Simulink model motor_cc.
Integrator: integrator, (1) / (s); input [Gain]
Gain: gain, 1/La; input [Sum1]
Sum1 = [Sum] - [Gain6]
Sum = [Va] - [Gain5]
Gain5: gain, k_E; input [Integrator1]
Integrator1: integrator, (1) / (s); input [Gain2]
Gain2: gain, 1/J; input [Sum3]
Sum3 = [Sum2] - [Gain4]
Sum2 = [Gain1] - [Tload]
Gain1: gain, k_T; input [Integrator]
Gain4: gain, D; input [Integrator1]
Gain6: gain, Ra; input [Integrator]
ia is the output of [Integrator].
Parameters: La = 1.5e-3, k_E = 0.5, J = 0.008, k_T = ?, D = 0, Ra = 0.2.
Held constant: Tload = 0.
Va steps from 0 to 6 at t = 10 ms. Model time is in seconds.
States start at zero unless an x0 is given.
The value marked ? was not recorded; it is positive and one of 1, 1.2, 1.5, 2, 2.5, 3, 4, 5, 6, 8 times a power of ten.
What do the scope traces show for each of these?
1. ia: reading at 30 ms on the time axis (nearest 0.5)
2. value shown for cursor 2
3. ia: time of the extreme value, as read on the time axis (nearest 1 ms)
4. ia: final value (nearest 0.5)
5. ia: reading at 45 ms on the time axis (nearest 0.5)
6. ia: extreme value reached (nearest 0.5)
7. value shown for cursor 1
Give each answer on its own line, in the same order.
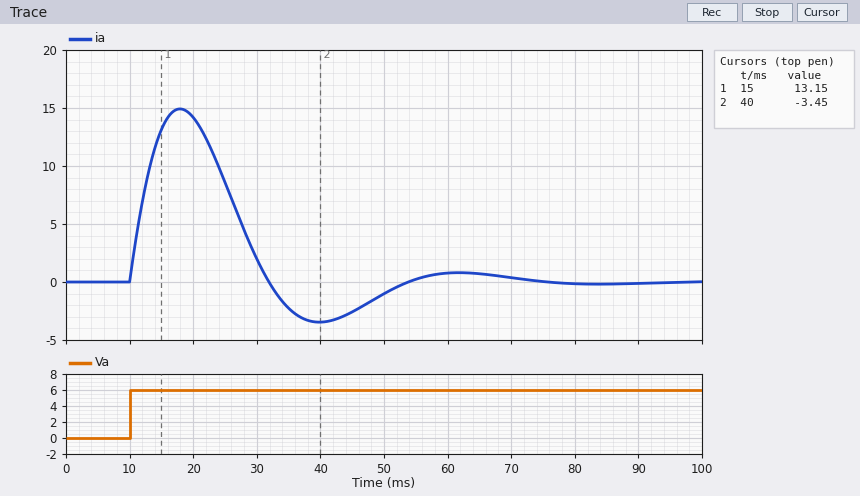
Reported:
2.0
-3.45
18 ms
0.0
-2.5
15.0
13.15
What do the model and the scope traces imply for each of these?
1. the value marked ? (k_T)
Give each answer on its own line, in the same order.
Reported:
0.6
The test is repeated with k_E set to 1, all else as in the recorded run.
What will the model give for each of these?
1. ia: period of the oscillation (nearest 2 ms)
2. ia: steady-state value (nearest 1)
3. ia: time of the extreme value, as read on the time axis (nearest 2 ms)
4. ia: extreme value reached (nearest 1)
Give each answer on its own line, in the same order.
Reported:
30 ms
0
16 ms
12
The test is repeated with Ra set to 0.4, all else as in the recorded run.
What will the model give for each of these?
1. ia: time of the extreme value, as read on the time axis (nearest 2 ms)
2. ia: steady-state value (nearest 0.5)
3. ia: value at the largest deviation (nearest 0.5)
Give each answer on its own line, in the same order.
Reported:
16 ms
0.0
10.5
